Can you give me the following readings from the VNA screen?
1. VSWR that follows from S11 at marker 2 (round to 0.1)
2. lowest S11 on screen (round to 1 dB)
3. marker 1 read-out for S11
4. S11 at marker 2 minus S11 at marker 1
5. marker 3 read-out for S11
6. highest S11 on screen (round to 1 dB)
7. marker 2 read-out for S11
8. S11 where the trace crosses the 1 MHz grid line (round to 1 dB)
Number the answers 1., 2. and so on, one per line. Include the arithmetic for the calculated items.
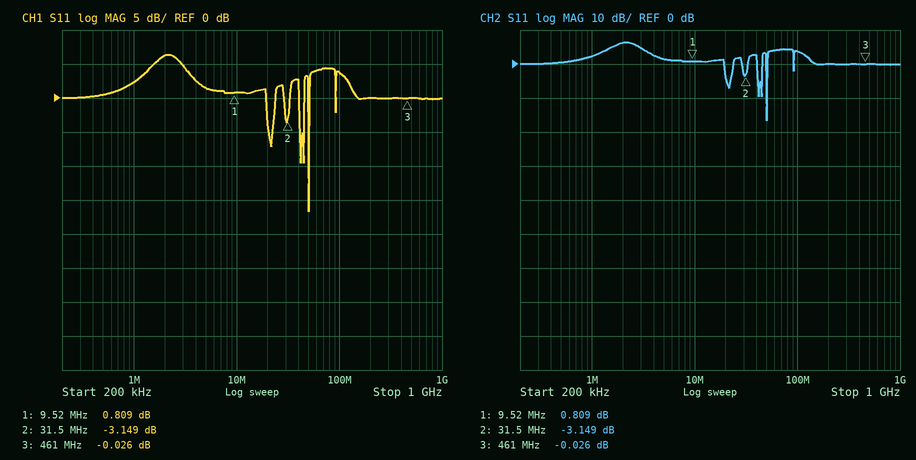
1. (1 + 0.6959)/(1 − 0.6959) ≈ 5.6
2. -17 dB
3. 0.809 dB
4. -3.149 − (0.809) = -3.958 dB
5. -0.026 dB
6. 6 dB
7. -3.149 dB
8. 2 dB
